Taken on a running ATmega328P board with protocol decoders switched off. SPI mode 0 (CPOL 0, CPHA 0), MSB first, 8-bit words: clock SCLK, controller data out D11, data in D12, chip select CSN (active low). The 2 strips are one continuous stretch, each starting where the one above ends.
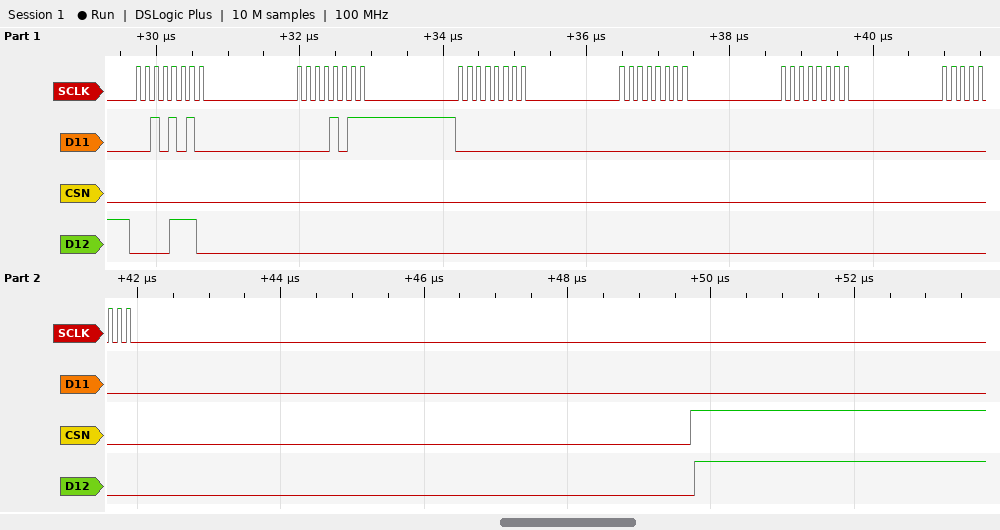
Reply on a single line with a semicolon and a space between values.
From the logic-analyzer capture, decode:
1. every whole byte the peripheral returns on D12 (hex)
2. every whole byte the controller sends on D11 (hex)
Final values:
0E 00 00 00 00 00; 2A 0B 00 00 00 00
